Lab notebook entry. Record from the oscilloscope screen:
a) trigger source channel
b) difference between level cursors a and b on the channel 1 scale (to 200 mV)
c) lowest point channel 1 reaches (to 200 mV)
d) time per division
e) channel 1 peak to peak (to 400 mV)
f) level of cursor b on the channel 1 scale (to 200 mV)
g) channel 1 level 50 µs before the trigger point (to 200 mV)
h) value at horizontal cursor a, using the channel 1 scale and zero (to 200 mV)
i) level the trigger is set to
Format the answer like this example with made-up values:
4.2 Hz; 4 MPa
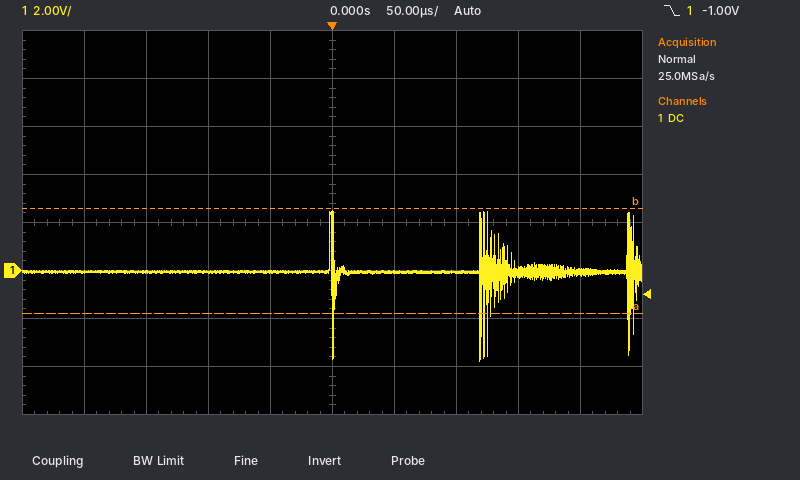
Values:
channel 1; 4.4 V; -3.8 V; 50 µs; 6.4 V; 2.6 V; 0.0 V; -1.8 V; -1.00 V
